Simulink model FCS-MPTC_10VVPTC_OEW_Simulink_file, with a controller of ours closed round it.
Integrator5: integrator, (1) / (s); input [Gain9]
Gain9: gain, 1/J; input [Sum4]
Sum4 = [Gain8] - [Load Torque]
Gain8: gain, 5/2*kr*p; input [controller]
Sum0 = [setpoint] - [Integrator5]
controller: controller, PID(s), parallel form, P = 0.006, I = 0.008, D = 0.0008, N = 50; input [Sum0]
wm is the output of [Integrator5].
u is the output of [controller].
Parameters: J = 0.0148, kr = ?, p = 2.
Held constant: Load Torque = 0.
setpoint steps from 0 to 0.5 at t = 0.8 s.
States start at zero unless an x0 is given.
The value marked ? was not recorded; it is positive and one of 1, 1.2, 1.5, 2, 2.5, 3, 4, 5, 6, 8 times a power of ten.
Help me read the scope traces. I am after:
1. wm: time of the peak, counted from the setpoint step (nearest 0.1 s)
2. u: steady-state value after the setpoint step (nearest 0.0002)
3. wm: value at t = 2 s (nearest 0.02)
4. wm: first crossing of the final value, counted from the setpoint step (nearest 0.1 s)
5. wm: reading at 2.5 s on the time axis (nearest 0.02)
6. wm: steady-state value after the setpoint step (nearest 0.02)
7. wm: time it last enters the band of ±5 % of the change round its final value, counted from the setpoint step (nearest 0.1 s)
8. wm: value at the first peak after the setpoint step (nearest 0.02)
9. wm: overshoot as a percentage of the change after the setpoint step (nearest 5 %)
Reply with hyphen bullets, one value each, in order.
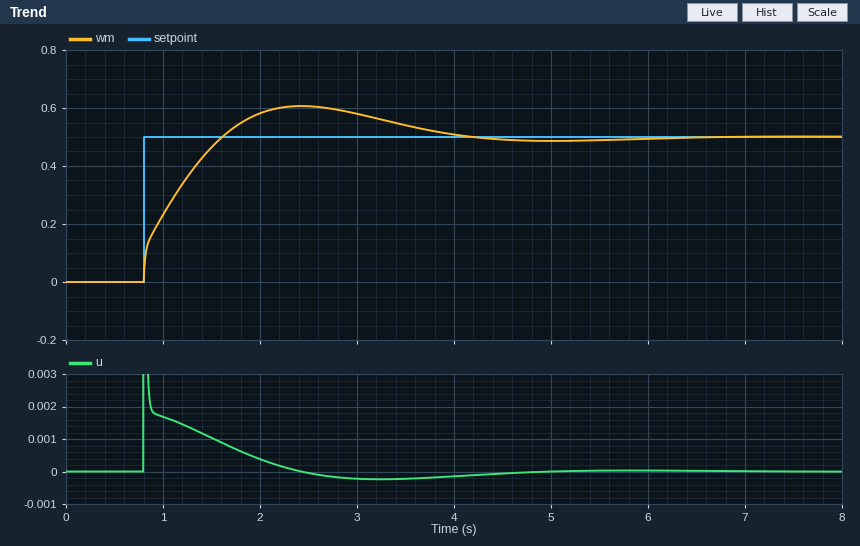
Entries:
- 1.6 s
- 0.0000
- 0.58
- 0.8 s
- 0.60
- 0.50
- 2.9 s
- 0.60
- 20 %
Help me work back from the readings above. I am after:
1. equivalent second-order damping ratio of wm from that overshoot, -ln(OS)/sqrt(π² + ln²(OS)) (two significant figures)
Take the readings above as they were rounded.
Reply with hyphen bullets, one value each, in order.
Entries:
- 0.46
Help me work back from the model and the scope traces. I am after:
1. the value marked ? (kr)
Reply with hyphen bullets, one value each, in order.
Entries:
- 1
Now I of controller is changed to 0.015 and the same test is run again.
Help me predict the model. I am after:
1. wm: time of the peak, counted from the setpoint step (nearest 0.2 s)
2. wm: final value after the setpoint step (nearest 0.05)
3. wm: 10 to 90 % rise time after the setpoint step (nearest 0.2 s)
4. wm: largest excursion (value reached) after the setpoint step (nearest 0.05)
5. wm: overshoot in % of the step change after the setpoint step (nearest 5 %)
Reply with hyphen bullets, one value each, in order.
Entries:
- 1.2 s
- 0.50
- 0.6 s
- 0.65
- 30 %
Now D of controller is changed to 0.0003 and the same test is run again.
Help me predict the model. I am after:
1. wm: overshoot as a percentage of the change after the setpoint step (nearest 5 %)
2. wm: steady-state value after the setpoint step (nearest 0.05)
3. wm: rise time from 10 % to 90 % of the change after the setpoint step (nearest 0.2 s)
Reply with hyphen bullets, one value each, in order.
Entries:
- 25 %
- 0.50
- 0.6 s
